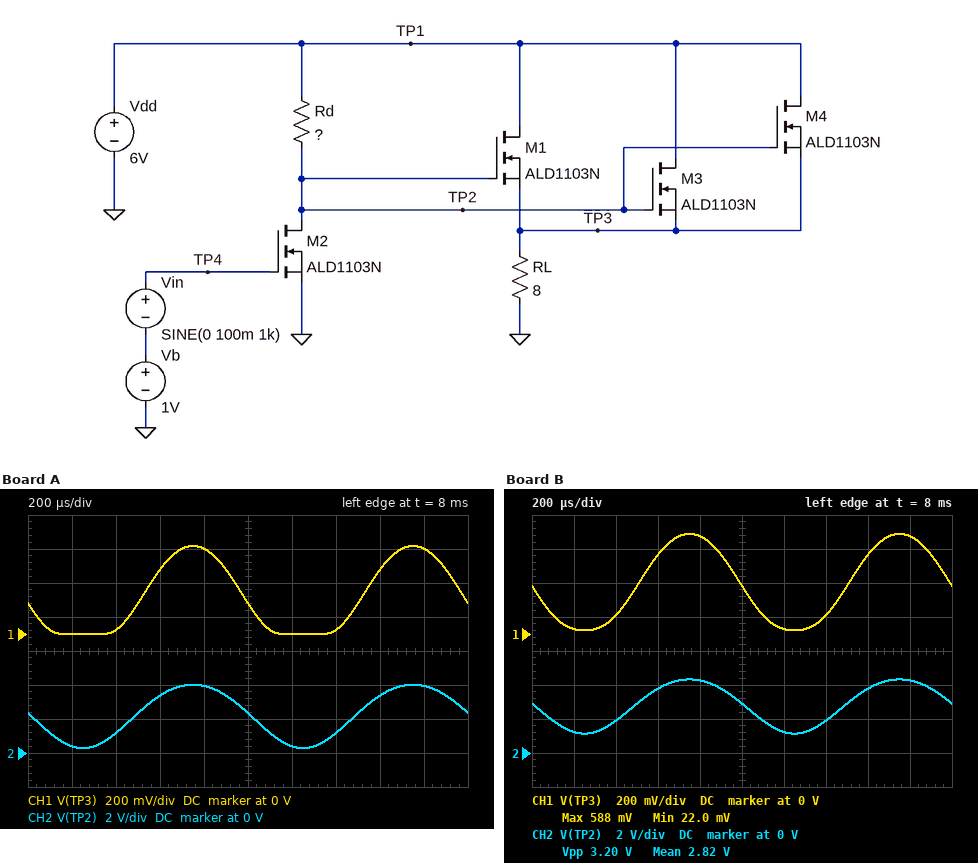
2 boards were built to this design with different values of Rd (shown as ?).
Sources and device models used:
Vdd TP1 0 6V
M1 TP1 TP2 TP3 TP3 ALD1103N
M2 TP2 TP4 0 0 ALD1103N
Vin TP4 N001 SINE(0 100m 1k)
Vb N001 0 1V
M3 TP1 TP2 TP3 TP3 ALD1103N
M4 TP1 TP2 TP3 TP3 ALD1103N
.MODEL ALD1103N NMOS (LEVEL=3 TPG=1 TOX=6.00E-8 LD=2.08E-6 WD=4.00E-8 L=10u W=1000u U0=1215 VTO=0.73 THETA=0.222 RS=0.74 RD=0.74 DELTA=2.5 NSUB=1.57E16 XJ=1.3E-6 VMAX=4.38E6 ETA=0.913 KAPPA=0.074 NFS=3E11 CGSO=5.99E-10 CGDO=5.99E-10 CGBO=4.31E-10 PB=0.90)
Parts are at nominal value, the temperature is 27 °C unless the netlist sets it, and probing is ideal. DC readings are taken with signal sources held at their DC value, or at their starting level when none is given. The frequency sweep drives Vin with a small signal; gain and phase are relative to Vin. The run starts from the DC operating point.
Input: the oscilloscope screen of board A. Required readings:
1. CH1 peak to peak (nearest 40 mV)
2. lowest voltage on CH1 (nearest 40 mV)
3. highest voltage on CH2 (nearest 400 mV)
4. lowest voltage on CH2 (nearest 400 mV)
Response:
520 mV
0 V
4.0 V
400 mV
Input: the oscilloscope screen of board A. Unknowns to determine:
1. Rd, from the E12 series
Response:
8.2 kΩ
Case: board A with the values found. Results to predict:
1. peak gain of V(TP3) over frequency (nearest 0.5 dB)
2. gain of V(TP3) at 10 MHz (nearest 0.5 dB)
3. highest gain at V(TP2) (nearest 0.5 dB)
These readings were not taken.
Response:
10.0 dB
-2.5 dB
25.5 dB
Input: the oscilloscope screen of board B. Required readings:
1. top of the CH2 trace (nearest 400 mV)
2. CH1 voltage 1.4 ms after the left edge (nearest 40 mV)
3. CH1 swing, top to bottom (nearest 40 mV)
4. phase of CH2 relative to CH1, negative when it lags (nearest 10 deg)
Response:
4.4 V
120 mV
560 mV
0 deg
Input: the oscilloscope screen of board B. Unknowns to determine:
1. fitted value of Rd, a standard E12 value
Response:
6.8 kΩ
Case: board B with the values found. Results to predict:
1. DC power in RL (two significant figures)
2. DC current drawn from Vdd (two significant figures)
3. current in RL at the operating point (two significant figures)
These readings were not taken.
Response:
10 mW
36 mA
35 mA
